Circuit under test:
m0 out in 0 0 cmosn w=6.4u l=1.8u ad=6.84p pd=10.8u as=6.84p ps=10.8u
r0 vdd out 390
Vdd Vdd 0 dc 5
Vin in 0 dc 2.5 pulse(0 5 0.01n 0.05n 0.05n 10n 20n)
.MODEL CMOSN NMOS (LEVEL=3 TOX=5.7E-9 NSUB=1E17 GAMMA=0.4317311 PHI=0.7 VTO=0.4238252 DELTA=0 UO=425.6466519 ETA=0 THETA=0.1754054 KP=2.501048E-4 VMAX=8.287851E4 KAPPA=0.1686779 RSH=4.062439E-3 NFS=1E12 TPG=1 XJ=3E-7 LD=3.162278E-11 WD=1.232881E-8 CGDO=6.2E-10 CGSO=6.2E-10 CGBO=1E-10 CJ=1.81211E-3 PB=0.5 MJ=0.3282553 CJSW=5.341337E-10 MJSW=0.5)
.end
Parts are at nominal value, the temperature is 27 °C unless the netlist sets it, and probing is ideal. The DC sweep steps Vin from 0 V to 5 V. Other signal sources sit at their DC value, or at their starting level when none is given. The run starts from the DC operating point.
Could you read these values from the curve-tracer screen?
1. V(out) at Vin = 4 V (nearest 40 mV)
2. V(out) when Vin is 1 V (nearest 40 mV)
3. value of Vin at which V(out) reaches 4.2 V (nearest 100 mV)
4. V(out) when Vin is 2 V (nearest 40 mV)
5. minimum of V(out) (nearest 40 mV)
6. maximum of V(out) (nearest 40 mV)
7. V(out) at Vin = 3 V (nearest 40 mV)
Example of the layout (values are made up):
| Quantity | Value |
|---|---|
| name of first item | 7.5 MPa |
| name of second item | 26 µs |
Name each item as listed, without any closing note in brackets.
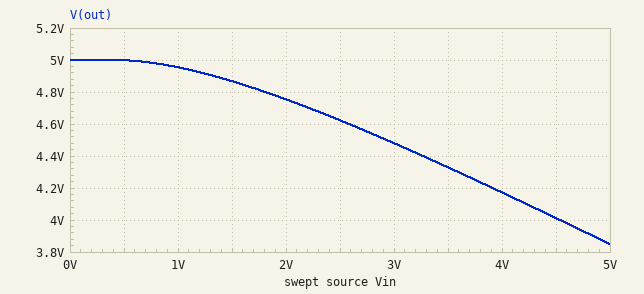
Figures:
| Quantity | Value |
|---|---|
| V(out) at Vin = 4 V | 4.16 V |
| V(out) when Vin is 1 V | 4.96 V |
| value of Vin at which V(out) reaches 4.2 V | 3.9 V |
| V(out) when Vin is 2 V | 4.76 V |
| minimum of V(out) | 3.84 V |
| maximum of V(out) | 5.00 V |
| V(out) at Vin = 3 V | 4.48 V |
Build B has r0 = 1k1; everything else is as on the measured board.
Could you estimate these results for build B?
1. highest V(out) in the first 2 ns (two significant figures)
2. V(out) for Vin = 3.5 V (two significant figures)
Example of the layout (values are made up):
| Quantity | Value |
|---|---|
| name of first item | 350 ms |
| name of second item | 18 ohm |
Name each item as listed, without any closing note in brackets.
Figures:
| Quantity | Value |
|---|---|
| highest V(out) in the first 2 ns | 5.2 V |
| V(out) for Vin = 3.5 V | 3.1 V |
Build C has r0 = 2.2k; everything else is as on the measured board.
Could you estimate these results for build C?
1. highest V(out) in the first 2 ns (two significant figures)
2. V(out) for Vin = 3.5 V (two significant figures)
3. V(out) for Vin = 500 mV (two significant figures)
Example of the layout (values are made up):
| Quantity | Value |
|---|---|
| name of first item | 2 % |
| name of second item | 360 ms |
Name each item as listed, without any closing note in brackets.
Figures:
| Quantity | Value |
|---|---|
| highest V(out) in the first 2 ns | 5.3 V |
| V(out) for Vin = 3.5 V | 1.6 V |
| V(out) for Vin = 500 mV | 5.0 V |
